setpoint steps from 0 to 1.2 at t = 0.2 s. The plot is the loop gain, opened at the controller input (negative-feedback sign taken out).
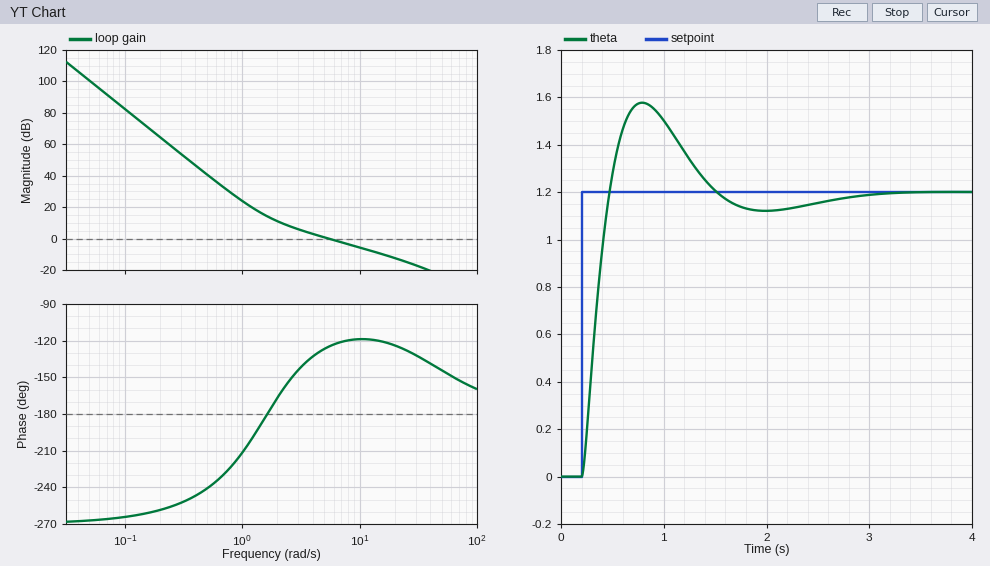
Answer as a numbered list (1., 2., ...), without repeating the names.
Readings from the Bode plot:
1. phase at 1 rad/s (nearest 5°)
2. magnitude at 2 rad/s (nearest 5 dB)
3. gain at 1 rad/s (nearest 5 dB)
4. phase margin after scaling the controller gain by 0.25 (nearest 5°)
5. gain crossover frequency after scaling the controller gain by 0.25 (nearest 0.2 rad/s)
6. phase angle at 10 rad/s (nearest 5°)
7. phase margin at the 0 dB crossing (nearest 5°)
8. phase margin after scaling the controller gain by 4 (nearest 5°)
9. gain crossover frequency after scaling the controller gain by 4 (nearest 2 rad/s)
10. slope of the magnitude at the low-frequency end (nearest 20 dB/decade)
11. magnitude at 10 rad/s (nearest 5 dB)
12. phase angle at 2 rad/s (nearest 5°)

1. -210°
2. 10 dB
3. 25 dB
4. 10°
5. 1.8 rad/s
6. -120°
7. 55°
8. 55°
9. 20 rad/s
10. -60 dB/decade
11. -5 dB
12. -165°
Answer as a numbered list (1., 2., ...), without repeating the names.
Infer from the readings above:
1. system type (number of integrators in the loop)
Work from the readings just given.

1. 3
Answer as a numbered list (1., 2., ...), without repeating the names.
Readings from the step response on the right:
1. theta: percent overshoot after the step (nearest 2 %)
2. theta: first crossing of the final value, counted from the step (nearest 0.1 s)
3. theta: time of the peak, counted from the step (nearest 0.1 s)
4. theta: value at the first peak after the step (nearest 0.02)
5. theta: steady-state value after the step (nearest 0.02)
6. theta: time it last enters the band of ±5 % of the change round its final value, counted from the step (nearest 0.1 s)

1. 32 %
2. 0.3 s
3. 0.6 s
4. 1.58
5. 1.20
6. 2.1 s
